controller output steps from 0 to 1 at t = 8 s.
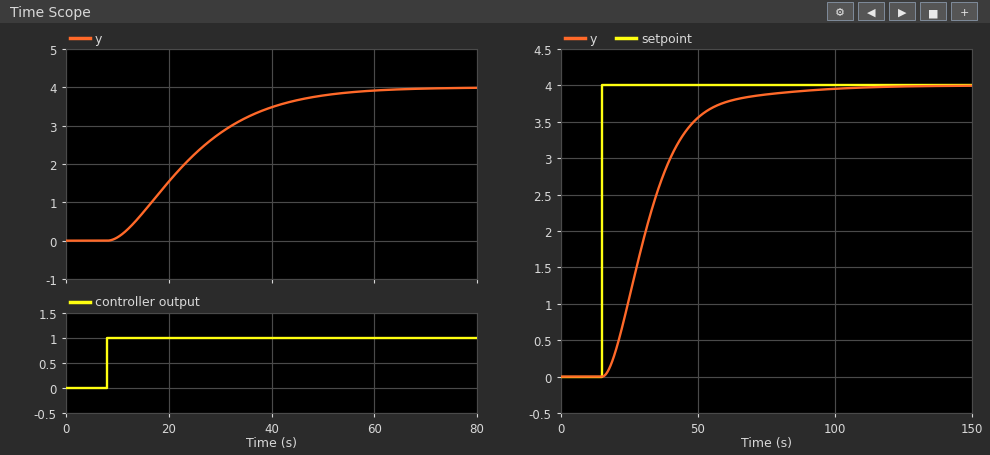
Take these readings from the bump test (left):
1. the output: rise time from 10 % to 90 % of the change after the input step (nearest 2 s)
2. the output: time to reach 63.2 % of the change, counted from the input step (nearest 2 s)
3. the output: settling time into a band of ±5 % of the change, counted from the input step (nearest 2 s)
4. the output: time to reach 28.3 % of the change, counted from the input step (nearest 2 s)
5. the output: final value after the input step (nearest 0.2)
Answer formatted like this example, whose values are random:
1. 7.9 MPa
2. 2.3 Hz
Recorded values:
1. 30 s
2. 20 s
3. 42 s
4. 10 s
5. 4.0
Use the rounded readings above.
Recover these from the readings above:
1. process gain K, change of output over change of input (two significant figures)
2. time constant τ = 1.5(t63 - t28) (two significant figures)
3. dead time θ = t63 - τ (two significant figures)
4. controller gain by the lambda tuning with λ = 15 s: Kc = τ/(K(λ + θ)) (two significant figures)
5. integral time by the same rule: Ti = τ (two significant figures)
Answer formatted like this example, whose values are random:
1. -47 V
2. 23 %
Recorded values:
1. 4.0
2. 15 s
3. 5.0 s
4. 0.19
5. 15 s
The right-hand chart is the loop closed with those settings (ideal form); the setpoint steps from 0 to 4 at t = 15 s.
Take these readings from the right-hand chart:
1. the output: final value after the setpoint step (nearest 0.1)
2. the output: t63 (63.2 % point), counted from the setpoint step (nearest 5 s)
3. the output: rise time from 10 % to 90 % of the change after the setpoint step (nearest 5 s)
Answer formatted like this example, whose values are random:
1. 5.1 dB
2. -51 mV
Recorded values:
1. 4.0
2. 20 s
3. 30 s
